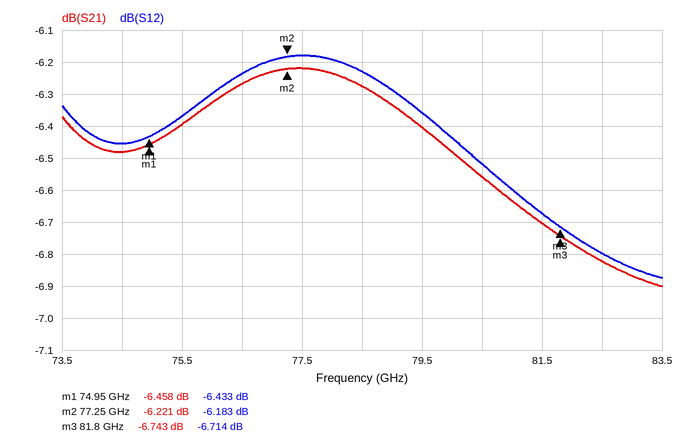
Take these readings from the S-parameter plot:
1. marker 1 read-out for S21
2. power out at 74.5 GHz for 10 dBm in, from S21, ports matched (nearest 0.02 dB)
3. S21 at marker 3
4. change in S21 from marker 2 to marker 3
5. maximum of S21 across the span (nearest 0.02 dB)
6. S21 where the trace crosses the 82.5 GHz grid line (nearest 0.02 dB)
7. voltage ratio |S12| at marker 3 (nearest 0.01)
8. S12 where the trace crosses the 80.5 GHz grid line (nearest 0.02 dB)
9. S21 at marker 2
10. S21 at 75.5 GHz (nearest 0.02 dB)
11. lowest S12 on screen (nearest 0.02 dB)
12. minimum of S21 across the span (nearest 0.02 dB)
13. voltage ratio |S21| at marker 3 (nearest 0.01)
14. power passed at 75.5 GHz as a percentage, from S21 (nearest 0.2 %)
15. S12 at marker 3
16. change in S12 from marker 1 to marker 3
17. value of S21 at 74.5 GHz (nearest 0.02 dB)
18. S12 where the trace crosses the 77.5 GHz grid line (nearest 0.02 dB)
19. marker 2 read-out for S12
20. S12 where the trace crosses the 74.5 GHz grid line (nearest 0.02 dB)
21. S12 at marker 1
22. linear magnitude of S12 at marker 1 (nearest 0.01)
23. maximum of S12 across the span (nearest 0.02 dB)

-6.458 dB
3.52 dBm
-6.743 dB
-0.522 dB
-6.22 dB
-6.82 dB
0.46
-6.52 dB
-6.221 dB
-6.40 dB
-6.88 dB
-6.90 dB
0.46
23.0 %
-6.714 dB
-0.281 dB
-6.48 dB
-6.18 dB
-6.183 dB
-6.46 dB
-6.433 dB
0.48
-6.18 dB
